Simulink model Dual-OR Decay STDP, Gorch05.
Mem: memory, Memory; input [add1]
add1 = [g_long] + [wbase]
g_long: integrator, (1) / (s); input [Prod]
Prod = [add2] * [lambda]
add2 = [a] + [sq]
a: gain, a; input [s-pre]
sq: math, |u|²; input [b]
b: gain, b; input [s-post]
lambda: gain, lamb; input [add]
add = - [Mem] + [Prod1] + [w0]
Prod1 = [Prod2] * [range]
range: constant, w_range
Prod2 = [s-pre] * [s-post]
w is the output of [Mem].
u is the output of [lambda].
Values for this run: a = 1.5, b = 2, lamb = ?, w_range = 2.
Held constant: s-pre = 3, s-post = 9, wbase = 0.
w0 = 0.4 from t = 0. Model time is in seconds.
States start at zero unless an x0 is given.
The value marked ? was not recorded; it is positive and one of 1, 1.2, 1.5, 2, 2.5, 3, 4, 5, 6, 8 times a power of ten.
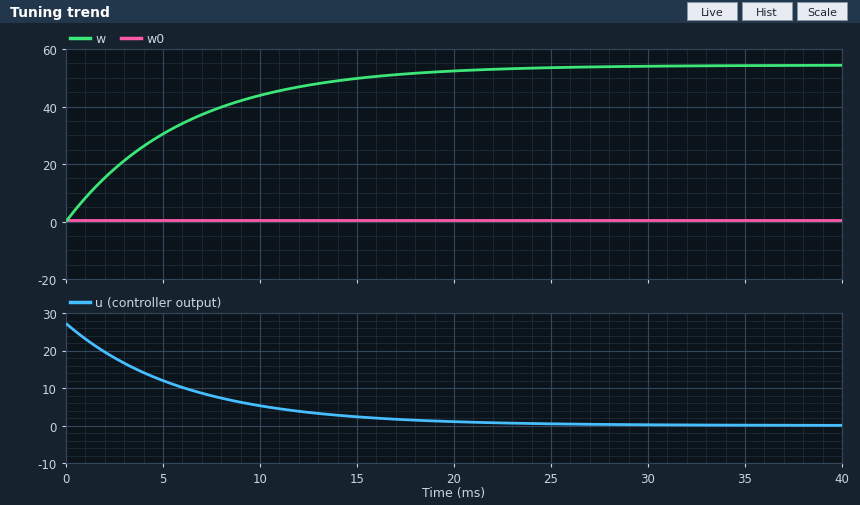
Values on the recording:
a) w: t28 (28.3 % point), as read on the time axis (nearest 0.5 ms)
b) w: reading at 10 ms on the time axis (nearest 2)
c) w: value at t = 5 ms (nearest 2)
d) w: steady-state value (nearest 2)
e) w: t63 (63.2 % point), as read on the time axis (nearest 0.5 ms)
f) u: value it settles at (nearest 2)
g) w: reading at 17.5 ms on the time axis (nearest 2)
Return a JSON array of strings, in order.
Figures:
["2.0 ms", "44", "30", "54", "6.0 ms", "0", "52"]
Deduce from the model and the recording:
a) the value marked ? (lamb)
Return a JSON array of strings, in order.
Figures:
["0.5"]
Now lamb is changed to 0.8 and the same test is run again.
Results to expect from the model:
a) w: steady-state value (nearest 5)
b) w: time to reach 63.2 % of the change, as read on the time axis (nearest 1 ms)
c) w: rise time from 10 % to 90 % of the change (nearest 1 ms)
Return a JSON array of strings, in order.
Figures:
["55", "4 ms", "8 ms"]
